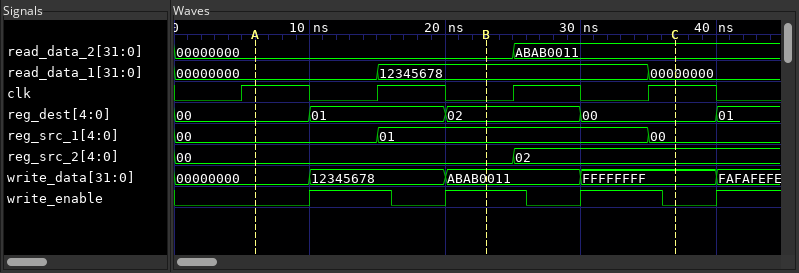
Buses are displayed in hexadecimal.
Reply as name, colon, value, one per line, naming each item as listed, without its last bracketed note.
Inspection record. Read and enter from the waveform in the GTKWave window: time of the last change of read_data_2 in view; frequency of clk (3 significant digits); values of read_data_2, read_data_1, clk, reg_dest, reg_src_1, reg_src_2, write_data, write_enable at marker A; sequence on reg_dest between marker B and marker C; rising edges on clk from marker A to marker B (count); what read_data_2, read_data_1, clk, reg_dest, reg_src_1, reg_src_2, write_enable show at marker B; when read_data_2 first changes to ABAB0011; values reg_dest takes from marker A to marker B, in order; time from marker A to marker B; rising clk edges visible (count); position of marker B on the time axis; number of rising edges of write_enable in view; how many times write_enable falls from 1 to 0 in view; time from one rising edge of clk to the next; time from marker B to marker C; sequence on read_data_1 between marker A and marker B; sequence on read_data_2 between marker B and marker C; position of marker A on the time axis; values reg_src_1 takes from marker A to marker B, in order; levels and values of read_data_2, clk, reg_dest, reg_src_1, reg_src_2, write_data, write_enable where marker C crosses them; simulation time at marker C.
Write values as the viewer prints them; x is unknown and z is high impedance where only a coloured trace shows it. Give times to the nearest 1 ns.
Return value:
time of the last change of read_data_2 in view: 25 ns
frequency of clk: 100 MHz
values of read_data_2, read_data_1, clk, reg_dest, reg_src_1, reg_src_2, write_data, write_enable at marker A: read_data_2=00000000, read_data_1=00000000, clk=1, reg_dest=00, reg_src_1=00, reg_src_2=00, write_data=00000000, write_enable=0
sequence on reg_dest between marker B and marker C: 02, 00
rising edges on clk from marker A to marker B: 1
what read_data_2, read_data_1, clk, reg_dest, reg_src_1, reg_src_2, write_enable show at marker B: read_data_2=00000000, read_data_1=12345678, clk=0, reg_dest=02, reg_src_1=01, reg_src_2=00, write_enable=1
when read_data_2 first changes to ABAB0011: 25 ns
values reg_dest takes from marker A to marker B, in order: 00, 01, 02
time from marker A to marker B: 17 ns
rising clk edges visible: 4
position of marker B on the time axis: 23 ns
number of rising edges of write_enable in view: 4
how many times write_enable falls from 1 to 0 in view: 3
time from one rising edge of clk to the next: 10 ns
time from marker B to marker C: 14 ns
sequence on read_data_1 between marker A and marker B: 00000000, 12345678
sequence on read_data_2 between marker B and marker C: 00000000, ABAB0011
position of marker A on the time axis: 6 ns
values reg_src_1 takes from marker A to marker B, in order: 00, 01
levels and values of read_data_2, clk, reg_dest, reg_src_1, reg_src_2, write_data, write_enable where marker C crosses them: read_data_2=ABAB0011, clk=1, reg_dest=00, reg_src_1=00, reg_src_2=02, write_data=FFFFFFFF, write_enable=0
simulation time at marker C: 37 ns
